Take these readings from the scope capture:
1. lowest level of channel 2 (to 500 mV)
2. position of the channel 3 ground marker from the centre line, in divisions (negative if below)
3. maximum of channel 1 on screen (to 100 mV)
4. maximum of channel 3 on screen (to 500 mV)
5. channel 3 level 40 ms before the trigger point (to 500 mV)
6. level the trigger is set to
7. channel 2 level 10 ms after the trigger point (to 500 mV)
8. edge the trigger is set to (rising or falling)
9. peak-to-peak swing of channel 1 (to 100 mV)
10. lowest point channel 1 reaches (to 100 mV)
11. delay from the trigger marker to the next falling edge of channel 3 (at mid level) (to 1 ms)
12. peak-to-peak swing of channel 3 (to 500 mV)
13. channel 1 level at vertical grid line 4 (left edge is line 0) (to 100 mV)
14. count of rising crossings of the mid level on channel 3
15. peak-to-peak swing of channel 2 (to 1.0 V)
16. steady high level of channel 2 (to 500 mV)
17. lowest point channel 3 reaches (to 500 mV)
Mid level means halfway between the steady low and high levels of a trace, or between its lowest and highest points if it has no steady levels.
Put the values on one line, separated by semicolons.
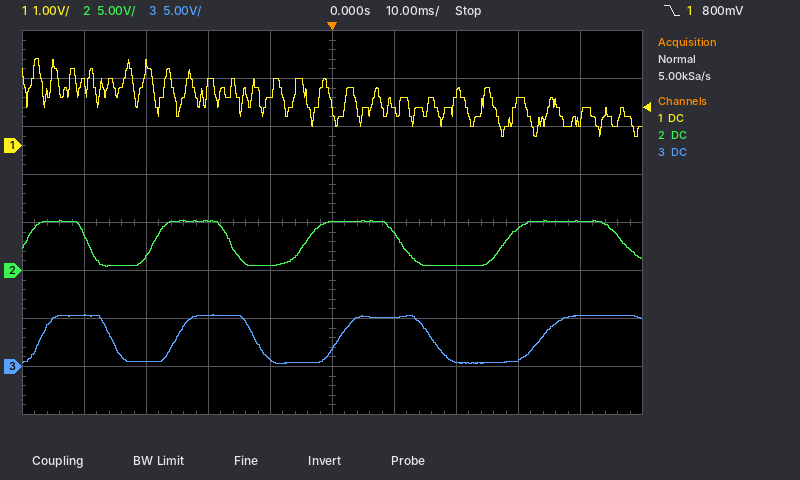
500 mV; -3.0 div; 1.8 V; 5.5 V; 5.5 V; 800 mV; 4.0 V; falling; 1.6 V; 200 mV; 16 ms; 5.0 V; 1.1 V; 4; 5.0 V; 5.0 V; 500 mV
